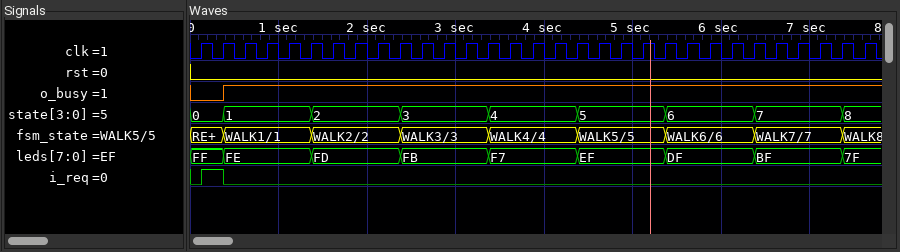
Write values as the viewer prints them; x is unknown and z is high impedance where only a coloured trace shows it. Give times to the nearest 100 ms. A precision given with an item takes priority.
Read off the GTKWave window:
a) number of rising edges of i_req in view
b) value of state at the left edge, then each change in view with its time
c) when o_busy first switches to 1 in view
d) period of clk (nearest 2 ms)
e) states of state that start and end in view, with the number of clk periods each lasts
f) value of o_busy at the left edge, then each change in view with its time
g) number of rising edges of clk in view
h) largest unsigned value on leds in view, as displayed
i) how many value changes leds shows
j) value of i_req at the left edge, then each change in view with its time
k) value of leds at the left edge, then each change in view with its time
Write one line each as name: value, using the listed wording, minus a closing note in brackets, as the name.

number of rising edges of i_req in view: 1
value of state at the left edge, then each change in view with its time: 0, 1 at 400 ms, 2 at 1400 ms, 3 at 2400 ms, 4 at 3400 ms, 5 at 4400 ms, 6 at 5400 ms, 7 at 6400 ms, 8 at 7400 ms
when o_busy first switches to 1 in view: 400 ms
period of clk: 250 ms
states of state that start and end in view, with the number of clk periods each lasts: 1: 4, 2: 4, 3: 4, 4: 4, 5: 4, 6: 4, 7: 4
value of o_busy at the left edge, then each change in view with its time: 0, 1 at 400 ms
number of rising edges of clk in view: 31
largest unsigned value on leds in view, as displayed: FF
how many value changes leds shows: 8
value of i_req at the left edge, then each change in view with its time: 0, 1 at 100 ms, 0 at 400 ms
value of leds at the left edge, then each change in view with its time: FF, FE at 400 ms, FD at 1400 ms, FB at 2400 ms, F7 at 3400 ms, EF at 4400 ms, DF at 5400 ms, BF at 6400 ms, 7F at 7400 ms
